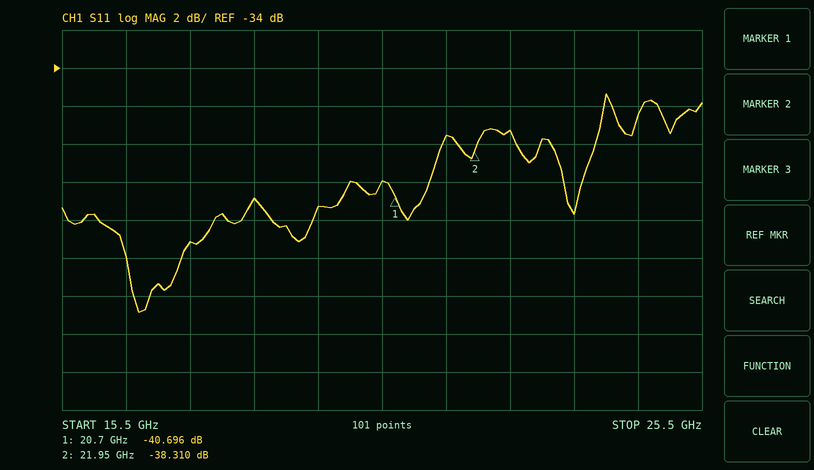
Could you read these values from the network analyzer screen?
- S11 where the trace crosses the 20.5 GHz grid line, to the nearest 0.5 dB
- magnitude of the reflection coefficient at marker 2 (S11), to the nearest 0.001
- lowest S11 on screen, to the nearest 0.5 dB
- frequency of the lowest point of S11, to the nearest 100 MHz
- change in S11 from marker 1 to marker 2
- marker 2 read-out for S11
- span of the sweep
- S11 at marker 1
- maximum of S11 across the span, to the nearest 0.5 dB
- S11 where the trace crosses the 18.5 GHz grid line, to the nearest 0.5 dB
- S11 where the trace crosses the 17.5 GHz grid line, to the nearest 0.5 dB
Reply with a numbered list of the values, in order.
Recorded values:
1. -40.0 dB
2. 0.012
3. -47.0 dB
4. 16.7 GHz
5. 2.386 dB
6. -38.310 dB
7. 10 GHz
8. -40.696 dB
9. -35.5 dB
10. -41.0 dB
11. -43.0 dB
